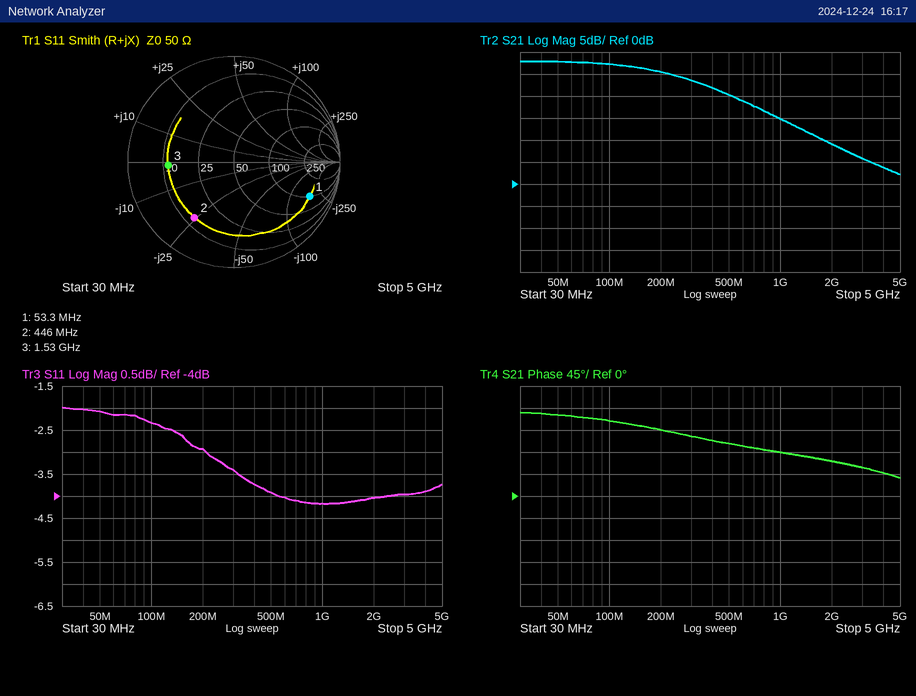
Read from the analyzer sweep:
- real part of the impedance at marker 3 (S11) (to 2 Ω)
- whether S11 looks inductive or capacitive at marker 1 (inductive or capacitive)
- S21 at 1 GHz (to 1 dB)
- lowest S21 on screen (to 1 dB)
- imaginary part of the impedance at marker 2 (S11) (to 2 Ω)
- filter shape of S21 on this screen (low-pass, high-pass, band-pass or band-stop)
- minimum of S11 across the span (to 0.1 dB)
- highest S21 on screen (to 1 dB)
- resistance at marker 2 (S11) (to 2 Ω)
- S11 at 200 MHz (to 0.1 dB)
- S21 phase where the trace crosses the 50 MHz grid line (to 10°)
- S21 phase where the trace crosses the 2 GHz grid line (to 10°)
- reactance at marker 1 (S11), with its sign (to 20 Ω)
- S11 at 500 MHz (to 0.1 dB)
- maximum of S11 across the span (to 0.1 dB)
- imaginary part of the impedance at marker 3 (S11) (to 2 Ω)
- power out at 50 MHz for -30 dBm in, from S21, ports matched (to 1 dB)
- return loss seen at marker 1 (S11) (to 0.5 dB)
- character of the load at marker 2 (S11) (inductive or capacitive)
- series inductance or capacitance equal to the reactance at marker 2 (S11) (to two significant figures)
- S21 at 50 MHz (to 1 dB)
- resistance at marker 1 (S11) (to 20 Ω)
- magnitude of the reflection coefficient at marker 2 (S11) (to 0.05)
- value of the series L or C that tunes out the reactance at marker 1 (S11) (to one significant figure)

12 Ω
capacitive
15 dB
2 dB
-24 Ω
low-pass
-4.2 dB
28 dB
14 Ω
-2.9 dB
170°
70°
-180 Ω
-3.9 dB
-2.0 dB
-2 Ω
-2 dBm
2.0 dB
capacitive
15 pF
28 dB
100 Ω
0.65
500 nH
